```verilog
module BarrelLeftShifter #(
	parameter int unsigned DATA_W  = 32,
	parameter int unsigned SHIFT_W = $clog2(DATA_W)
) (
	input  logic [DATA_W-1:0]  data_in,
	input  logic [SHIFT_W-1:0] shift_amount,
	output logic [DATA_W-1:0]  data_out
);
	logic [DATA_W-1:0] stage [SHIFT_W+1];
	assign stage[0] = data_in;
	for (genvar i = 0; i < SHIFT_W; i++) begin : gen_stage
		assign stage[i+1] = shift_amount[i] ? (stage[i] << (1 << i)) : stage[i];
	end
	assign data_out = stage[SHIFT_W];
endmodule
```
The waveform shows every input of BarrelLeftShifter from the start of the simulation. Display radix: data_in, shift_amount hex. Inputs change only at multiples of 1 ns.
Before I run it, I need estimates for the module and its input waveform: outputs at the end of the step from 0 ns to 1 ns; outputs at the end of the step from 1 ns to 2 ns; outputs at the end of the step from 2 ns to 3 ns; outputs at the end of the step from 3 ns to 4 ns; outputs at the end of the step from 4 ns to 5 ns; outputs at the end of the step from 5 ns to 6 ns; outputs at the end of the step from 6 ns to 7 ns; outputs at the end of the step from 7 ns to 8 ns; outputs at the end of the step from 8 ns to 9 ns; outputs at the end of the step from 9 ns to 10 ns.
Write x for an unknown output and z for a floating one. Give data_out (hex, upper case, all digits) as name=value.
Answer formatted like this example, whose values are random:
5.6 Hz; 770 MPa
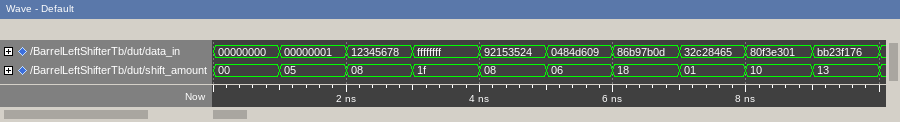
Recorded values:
data_out=00000000; data_out=00000020; data_out=34567800; data_out=80000000; data_out=15352400; data_out=21358240; data_out=0D000000; data_out=658508CA; data_out=E3010000; data_out=8BB00000
